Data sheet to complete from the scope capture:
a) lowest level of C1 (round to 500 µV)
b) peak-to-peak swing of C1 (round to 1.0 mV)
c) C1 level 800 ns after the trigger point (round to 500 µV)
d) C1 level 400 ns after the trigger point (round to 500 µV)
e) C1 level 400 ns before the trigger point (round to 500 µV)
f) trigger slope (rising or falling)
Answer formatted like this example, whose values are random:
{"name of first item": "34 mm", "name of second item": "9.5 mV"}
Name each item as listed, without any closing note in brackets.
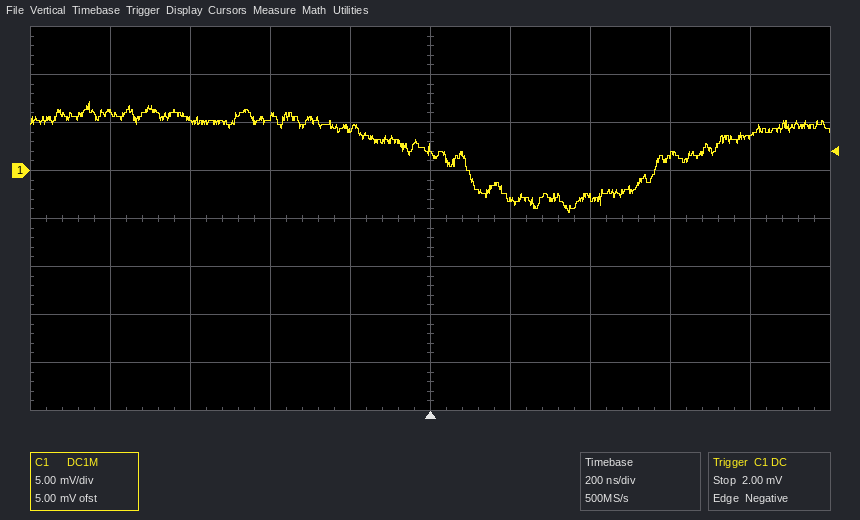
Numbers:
{"lowest level of C1": "-4.5 mV", "peak-to-peak swing of C1": "12.0 mV", "C1 level 800 ns after the trigger point": "3.5 mV", "C1 level 400 ns after the trigger point": "-3.0 mV", "C1 level 400 ns before the trigger point": "5.5 mV", "trigger slope": "falling"}
